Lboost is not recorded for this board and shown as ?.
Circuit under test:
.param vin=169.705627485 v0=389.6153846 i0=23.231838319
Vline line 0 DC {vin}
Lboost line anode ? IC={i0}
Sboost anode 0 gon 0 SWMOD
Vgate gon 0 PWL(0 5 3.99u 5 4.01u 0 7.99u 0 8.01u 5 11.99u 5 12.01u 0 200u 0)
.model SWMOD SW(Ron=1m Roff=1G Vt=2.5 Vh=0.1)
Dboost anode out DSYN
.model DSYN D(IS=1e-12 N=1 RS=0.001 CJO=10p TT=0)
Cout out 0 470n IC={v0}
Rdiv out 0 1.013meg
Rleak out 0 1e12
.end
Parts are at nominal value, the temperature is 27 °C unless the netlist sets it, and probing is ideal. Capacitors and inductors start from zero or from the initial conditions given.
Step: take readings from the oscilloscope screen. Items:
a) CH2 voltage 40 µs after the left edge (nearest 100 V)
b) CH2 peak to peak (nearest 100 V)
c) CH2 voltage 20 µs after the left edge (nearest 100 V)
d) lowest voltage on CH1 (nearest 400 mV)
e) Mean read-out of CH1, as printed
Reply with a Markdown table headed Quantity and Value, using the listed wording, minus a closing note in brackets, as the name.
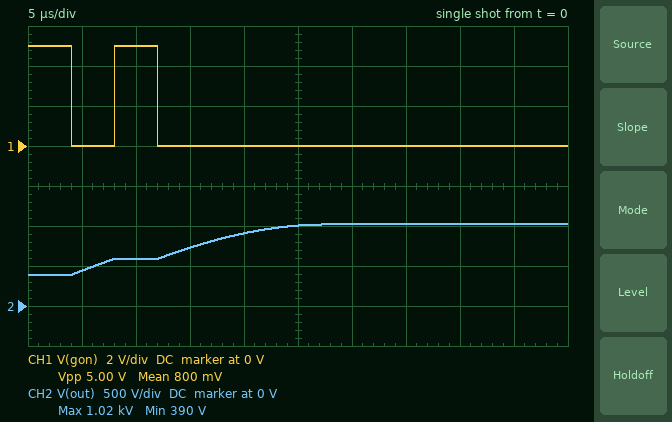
| Quantity | Value |
|---|---|
| CH2 voltage 40 µs after the left edge | 1.0 kV |
| CH2 peak to peak | 600 V |
| CH2 voltage 20 µs after the left edge | 900 V |
| lowest voltage on CH1 | 0 V |
| Mean read-out of CH1, as printed | 800 mV |
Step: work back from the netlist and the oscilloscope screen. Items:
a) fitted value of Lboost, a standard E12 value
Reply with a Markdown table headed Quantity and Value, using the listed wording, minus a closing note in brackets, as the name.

| Quantity | Value |
|---|---|
| fitted value of Lboost, a standard E12 value | 470 µH |
